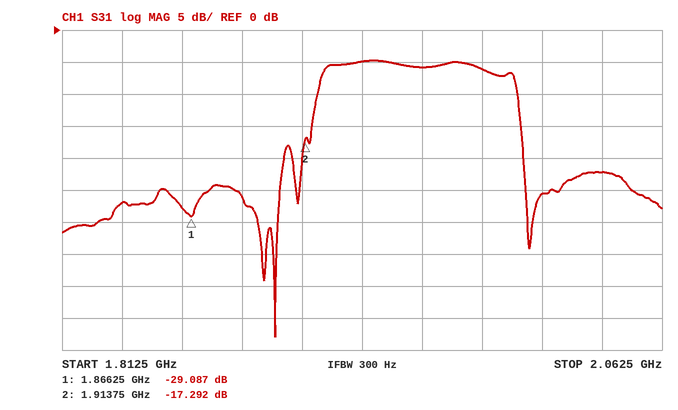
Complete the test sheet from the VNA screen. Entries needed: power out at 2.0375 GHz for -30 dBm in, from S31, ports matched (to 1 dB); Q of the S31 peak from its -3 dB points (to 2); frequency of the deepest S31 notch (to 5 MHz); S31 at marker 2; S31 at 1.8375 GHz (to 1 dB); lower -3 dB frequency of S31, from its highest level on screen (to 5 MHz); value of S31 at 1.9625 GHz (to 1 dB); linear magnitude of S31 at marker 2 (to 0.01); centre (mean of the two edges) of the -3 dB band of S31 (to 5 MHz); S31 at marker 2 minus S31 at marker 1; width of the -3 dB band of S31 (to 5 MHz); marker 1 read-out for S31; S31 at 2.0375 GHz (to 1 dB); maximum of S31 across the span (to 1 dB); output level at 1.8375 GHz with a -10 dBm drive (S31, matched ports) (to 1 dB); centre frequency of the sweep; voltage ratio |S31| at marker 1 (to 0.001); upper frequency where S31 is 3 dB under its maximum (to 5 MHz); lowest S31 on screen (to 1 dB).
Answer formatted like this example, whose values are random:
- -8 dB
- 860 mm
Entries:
- -52 dBm
- 24
- 1.900 GHz
- -17.292 dB
- -27 dB
- 1.920 GHz
- -6 dB
- 0.14
- 1.960 GHz
- 11.795 dB
- 80 MHz
- -29.087 dB
- -22 dB
- -5 dB
- -37 dBm
- 1.9375 GHz
- 0.035
- 2.000 GHz
- -48 dB
